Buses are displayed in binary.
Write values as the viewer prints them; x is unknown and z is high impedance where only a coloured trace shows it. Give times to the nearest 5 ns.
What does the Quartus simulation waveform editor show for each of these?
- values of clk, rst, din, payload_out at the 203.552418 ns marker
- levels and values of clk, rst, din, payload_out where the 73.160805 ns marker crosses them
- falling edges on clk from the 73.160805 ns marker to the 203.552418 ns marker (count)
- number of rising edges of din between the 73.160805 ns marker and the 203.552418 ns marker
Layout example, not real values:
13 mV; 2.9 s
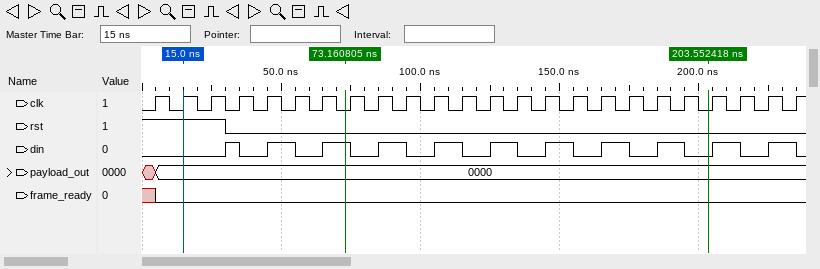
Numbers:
clk=0, rst=0, din=0, payload_out=0000; clk=0, rst=0, din=1, payload_out=0000; 13; 6
